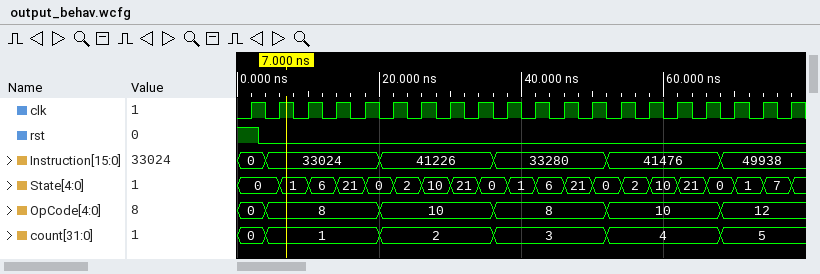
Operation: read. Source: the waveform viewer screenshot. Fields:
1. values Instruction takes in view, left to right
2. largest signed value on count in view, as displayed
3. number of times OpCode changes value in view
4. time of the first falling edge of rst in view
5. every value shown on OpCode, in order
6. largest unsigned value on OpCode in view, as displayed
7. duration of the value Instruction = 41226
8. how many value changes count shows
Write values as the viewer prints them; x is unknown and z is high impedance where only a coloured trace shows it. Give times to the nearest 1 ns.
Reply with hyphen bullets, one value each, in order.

- 0, 33024, 41226, 33280, 41476, 49938
- 5
- 5
- 3 ns
- 0, 8, 10, 8, 10, 12
- 12
- 16 ns
- 5
